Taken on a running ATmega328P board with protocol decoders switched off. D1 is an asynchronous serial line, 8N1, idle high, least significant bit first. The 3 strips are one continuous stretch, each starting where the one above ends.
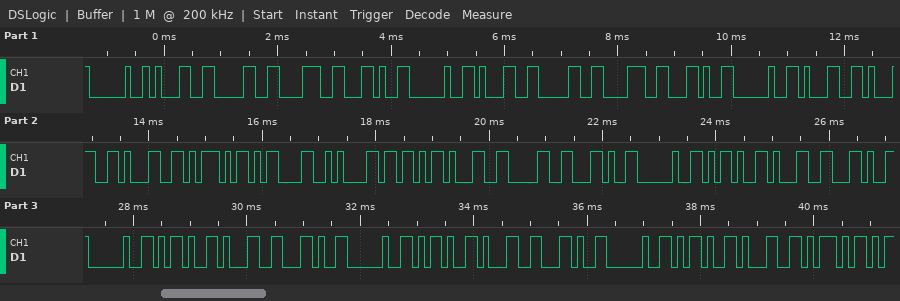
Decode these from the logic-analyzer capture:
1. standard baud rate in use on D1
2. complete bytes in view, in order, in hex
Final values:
9600 baud
20 31 30 38 2C 20 31 30 38 2C 20 31 31 31 5D 0D 0A 5B 31 30 2C 20 2D 31 2C 20 2D 31 2C 20 2D 31 2C 20 2D 31 5D
